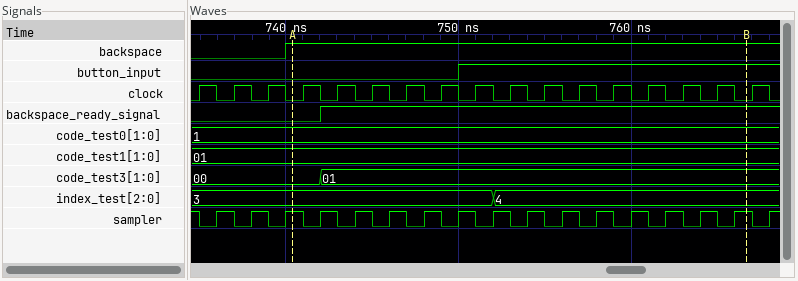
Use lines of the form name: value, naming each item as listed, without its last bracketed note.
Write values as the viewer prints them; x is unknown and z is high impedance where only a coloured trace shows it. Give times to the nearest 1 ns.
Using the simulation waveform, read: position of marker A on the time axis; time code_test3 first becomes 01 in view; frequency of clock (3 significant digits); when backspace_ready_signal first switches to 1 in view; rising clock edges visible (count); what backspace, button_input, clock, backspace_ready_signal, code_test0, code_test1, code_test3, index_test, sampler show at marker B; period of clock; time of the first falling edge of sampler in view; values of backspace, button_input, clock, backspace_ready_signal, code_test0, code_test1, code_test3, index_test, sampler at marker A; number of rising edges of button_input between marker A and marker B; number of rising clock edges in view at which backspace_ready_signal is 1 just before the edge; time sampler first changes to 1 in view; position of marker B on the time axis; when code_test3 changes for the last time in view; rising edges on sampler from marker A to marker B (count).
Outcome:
position of marker A on the time axis: 740 ns
time code_test3 first becomes 01 in view: 742 ns
frequency of clock: 500 MHz
when backspace_ready_signal first switches to 1 in view: 742 ns
rising clock edges visible: 17
what backspace, button_input, clock, backspace_ready_signal, code_test0, code_test1, code_test3, index_test, sampler show at marker B: backspace=1, button_input=1, clock=0, backspace_ready_signal=1, code_test0=1, code_test1=01, code_test3=01, index_test=4, sampler=1
period of clock: 2 ns
time of the first falling edge of sampler in view: 735 ns
values of backspace, button_input, clock, backspace_ready_signal, code_test0, code_test1, code_test3, index_test, sampler at marker A: backspace=1, button_input=0, clock=0, backspace_ready_signal=0, code_test0=1, code_test1=01, code_test3=00, index_test=3, sampler=1
number of rising edges of button_input between marker A and marker B: 1
number of rising clock edges in view at which backspace_ready_signal is 1 just before the edge: 13
time sampler first changes to 1 in view: 736 ns
position of marker B on the time axis: 767 ns
when code_test3 changes for the last time in view: 742 ns
rising edges on sampler from marker A to marker B: 13
